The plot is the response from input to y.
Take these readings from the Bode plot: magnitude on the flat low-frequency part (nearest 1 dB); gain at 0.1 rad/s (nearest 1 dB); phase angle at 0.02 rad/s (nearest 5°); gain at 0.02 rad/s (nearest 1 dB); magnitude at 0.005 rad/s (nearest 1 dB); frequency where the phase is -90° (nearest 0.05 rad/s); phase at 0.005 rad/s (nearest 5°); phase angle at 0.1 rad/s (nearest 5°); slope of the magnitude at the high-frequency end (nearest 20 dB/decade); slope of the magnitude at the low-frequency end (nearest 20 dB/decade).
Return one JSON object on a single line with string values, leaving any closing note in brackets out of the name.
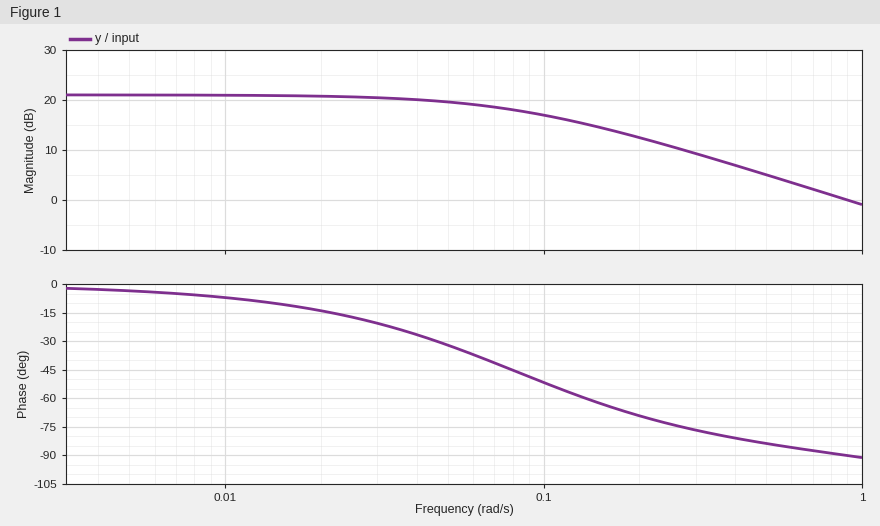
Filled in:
{"magnitude on the flat low-frequency part": "21 dB", "gain at 0.1 rad/s": "17 dB", "phase angle at 0.02 rad/s": "-15°", "gain at 0.02 rad/s": "21 dB", "magnitude at 0.005 rad/s": "21 dB", "frequency where the phase is -90°": "0.90 rad/s", "phase at 0.005 rad/s": "-5°", "phase angle at 0.1 rad/s": "-50°", "slope of the magnitude at the high-frequency end": "-20 dB/decade", "slope of the magnitude at the low-frequency end": "0 dB/decade"}
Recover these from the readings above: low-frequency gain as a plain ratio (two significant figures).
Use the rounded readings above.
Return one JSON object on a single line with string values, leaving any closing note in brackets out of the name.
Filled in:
{"low-frequency gain as a plain ratio": "11"}
